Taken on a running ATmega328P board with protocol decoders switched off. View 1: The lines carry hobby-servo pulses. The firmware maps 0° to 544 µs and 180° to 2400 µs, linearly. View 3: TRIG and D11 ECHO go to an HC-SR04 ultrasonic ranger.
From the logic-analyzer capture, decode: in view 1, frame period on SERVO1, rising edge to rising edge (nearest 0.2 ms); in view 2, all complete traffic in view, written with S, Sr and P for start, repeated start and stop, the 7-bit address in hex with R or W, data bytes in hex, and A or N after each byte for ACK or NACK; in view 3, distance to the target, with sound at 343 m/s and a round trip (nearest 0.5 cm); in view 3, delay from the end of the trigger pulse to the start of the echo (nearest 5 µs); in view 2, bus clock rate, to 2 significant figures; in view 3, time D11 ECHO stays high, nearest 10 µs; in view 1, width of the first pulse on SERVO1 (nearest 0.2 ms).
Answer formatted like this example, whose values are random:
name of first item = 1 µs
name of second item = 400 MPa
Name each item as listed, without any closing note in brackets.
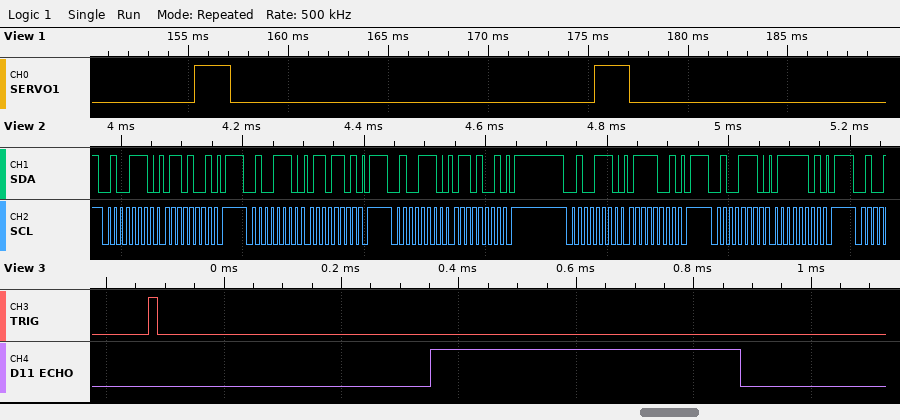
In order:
in view 1, frame period on SERVO1, rising edge to rising edge = 20.0 ms
in view 2, all complete traffic in view, written with S, Sr and P for start, repeated start and stop, the 7-bit address in hex with R or W, data bytes in hex, and A or N after each byte for ACK or NACK = S 27W A 69 A P S 27W A 6D A P S 27W A 69 A P S 27W A 79 A P S 27W A 7D A P
in view 3, distance to the target, with sound at 343 m/s and a round trip = 9 cm
in view 3, delay from the end of the trigger pulse to the start of the echo = 465 µs
in view 2, bus clock rate, to 2 significant figures = 100 kHz
in view 3, time D11 ECHO stays high, nearest 10 µs = 530 µs
in view 1, width of the first pulse on SERVO1 = 1.8 ms
